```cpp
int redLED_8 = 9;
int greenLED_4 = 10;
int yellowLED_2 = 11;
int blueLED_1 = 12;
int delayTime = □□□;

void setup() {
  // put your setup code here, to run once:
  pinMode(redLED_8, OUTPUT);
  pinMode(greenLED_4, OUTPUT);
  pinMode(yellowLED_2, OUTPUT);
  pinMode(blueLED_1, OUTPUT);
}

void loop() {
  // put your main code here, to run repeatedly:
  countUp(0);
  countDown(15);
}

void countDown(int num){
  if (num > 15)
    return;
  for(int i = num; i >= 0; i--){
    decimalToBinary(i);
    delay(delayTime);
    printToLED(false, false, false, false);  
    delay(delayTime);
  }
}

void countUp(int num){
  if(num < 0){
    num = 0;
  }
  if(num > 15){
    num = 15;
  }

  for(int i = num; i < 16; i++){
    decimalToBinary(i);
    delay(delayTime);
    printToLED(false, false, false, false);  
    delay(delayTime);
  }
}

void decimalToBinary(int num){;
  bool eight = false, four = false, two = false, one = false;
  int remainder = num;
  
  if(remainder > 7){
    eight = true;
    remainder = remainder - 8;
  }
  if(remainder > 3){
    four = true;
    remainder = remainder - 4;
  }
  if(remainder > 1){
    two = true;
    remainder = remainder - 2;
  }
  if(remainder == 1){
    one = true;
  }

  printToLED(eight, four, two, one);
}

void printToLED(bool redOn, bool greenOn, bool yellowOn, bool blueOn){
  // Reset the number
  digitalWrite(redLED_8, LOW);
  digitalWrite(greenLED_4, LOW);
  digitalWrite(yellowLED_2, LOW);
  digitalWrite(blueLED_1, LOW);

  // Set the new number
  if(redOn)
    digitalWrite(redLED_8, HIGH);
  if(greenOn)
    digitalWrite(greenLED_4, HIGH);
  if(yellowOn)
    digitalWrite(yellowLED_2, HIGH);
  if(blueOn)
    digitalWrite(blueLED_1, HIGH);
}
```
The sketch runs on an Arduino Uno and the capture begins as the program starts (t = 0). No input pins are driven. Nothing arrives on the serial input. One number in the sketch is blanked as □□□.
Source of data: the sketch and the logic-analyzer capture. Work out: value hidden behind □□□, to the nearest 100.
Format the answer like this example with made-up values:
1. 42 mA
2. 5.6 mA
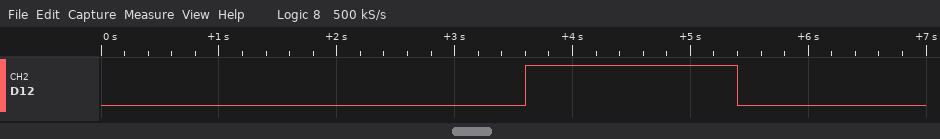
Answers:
1. 1800
